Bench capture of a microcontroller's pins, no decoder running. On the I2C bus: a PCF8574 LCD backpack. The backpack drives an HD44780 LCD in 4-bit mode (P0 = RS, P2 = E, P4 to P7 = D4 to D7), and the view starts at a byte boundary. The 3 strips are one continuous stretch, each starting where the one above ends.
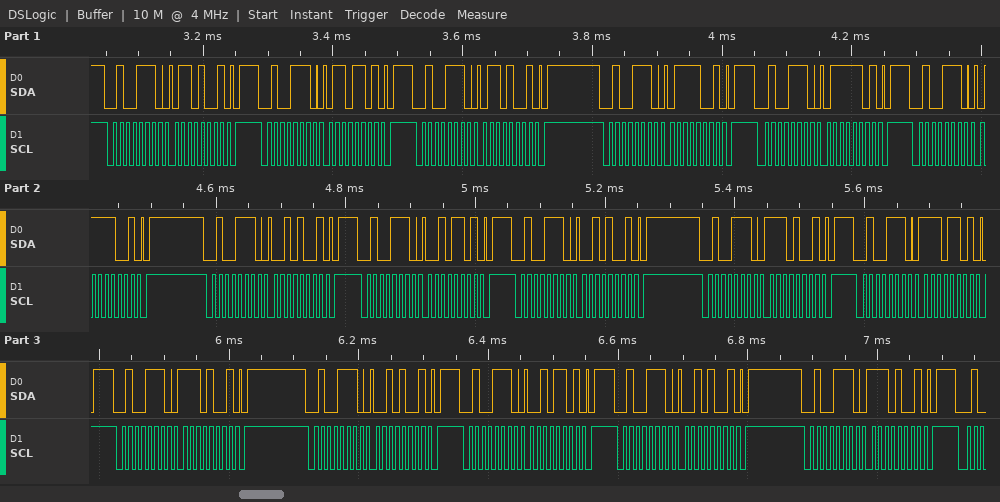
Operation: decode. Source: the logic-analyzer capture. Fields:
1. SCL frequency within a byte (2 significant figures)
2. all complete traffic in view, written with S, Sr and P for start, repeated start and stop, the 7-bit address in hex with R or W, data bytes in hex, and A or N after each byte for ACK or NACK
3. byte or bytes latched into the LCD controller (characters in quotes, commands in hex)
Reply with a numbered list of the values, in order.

1. 100 kHz
2. S 27W A 69 A P S 27W A 6D A P S 27W A 69 A P S 27W A 79 A P S 27W A 7D A P S 27W A 79 A P S 27W A 29 A P S 27W A 2D A P S 27W A 29 A P S 27W A E9 A P S 27W A ED A P S 27W A E9 A P S 27W A 29 A P S 27W A 2D A P S 27W A 29 A P S 27W A E9 A P
3. 'g' '.'
